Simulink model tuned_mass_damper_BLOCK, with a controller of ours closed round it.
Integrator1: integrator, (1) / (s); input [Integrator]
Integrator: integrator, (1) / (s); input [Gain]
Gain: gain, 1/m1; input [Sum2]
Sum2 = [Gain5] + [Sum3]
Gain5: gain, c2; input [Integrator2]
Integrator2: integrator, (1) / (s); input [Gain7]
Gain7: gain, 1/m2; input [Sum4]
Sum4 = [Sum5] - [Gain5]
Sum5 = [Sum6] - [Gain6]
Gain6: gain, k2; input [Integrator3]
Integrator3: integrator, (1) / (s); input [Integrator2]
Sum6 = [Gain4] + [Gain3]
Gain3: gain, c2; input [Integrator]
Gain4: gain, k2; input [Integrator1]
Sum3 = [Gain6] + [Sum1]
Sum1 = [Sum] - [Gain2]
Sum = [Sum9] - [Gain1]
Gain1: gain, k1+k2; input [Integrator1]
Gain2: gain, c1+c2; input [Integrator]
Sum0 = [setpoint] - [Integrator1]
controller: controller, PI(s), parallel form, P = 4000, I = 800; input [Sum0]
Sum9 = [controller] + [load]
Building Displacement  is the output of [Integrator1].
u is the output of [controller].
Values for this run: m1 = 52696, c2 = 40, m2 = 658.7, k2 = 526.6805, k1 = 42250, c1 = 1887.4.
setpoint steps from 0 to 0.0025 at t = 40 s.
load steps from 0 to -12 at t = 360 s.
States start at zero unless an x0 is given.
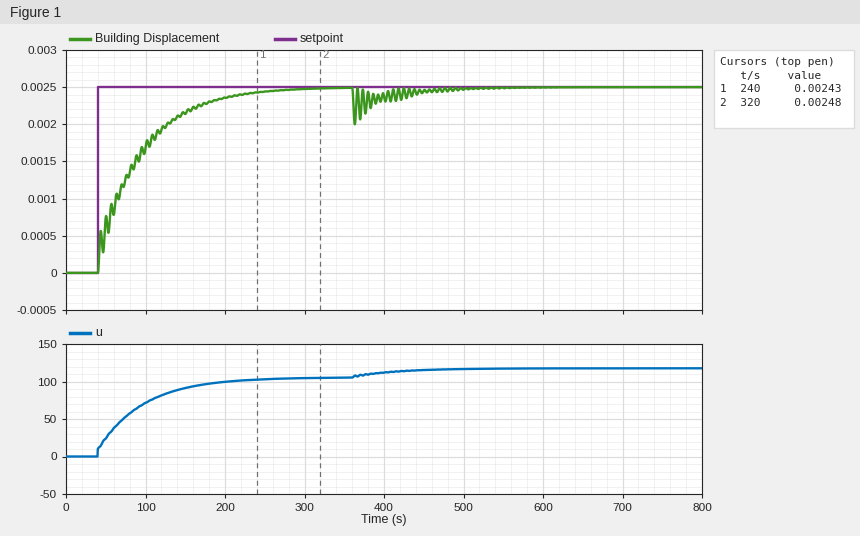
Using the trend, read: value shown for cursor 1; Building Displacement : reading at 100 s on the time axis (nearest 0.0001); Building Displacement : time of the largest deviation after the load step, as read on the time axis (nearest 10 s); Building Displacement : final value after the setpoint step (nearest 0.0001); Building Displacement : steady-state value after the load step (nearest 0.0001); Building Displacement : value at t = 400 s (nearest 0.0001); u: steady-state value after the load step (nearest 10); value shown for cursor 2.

0.00243
0.0017
360 s
0.0025
0.0025
0.0024
120
0.00248
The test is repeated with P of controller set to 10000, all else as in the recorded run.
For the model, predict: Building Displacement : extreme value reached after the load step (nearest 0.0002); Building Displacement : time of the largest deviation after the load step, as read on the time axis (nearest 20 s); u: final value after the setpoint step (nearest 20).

0.0020
360 s
100
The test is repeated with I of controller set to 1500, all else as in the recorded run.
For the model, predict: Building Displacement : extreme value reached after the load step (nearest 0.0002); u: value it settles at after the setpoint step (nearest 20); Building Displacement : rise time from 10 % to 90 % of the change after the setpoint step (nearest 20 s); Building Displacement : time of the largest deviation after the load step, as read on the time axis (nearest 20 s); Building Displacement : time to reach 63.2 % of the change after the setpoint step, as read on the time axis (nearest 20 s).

0.0020
100
60 s
360 s
60 s
